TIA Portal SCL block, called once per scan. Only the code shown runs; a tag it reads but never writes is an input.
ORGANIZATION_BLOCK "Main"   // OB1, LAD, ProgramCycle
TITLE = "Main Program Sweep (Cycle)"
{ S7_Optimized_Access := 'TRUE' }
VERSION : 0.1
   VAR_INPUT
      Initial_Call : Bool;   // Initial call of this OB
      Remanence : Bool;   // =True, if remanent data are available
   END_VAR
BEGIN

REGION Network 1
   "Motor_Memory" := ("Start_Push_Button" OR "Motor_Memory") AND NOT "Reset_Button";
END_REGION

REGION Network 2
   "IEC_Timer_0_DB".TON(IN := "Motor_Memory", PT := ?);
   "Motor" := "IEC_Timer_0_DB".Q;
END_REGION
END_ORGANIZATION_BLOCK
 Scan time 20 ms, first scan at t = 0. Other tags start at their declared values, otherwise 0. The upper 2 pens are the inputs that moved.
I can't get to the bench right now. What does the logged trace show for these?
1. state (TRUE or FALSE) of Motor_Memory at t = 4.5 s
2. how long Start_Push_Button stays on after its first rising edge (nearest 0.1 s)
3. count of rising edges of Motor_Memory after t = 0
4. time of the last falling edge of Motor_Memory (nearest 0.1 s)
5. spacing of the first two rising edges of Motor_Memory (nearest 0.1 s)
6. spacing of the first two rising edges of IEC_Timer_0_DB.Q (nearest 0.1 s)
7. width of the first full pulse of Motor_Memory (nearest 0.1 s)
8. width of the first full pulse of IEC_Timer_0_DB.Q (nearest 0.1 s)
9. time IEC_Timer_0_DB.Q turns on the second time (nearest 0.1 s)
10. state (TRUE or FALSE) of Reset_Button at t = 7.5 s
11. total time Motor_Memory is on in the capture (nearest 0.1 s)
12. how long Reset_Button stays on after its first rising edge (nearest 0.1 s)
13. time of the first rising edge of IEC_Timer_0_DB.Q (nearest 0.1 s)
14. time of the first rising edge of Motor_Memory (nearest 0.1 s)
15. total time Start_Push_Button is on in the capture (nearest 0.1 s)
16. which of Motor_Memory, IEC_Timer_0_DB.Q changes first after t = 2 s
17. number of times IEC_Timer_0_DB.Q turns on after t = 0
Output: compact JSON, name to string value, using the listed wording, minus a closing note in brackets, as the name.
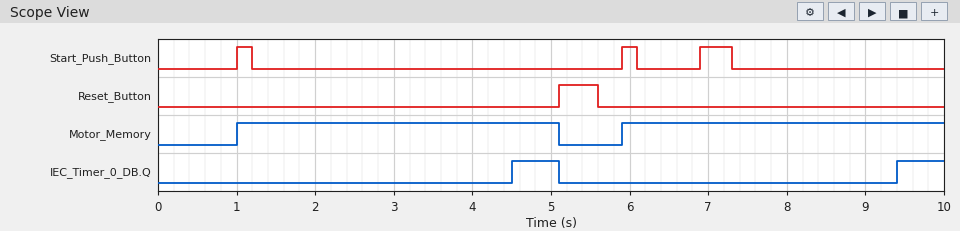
{"state (TRUE or FALSE) of Motor_Memory at t = 4.5 s": "TRUE", "how long Start_Push_Button stays on after its first rising edge": "0.2 s", "count of rising edges of Motor_Memory after t = 0": "2", "time of the last falling edge of Motor_Memory": "5.1 s", "spacing of the first two rising edges of Motor_Memory": "4.9 s", "spacing of the first two rising edges of IEC_Timer_0_DB.Q": "4.9 s", "width of the first full pulse of Motor_Memory": "4.1 s", "width of the first full pulse of IEC_Timer_0_DB.Q": "0.6 s", "time IEC_Timer_0_DB.Q turns on the second time": "9.4 s", "state (TRUE or FALSE) of Reset_Button at t = 7.5 s": "FALSE", "total time Motor_Memory is on in the capture": "8.2 s", "how long Reset_Button stays on after its first rising edge": "0.5 s", "time of the first rising edge of IEC_Timer_0_DB.Q": "4.5 s", "time of the first rising edge of Motor_Memory": "1.0 s", "total time Start_Push_Button is on in the capture": "0.8 s", "which of Motor_Memory, IEC_Timer_0_DB.Q changes first after t = 2 s": "IEC_Timer_0_DB.Q", "number of times IEC_Timer_0_DB.Q turns on after t = 0": "2"}
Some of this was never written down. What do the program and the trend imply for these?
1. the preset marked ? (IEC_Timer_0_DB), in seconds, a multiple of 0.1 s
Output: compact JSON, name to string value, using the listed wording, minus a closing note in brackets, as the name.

{"the preset marked ? (IEC_Timer_0_DB), in seconds, a multiple of 0.1 s": "3.5 s"}
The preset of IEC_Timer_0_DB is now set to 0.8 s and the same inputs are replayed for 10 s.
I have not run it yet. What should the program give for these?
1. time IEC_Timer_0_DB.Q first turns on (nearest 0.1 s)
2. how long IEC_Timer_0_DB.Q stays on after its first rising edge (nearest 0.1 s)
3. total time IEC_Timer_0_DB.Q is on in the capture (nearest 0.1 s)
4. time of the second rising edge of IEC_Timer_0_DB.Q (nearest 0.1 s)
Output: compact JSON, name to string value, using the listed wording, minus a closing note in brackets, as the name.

{"time IEC_Timer_0_DB.Q first turns on": "1.8 s", "how long IEC_Timer_0_DB.Q stays on after its first rising edge": "3.3 s", "total time IEC_Timer_0_DB.Q is on in the capture": "6.6 s", "time of the second rising edge of IEC_Timer_0_DB.Q": "6.7 s"}
